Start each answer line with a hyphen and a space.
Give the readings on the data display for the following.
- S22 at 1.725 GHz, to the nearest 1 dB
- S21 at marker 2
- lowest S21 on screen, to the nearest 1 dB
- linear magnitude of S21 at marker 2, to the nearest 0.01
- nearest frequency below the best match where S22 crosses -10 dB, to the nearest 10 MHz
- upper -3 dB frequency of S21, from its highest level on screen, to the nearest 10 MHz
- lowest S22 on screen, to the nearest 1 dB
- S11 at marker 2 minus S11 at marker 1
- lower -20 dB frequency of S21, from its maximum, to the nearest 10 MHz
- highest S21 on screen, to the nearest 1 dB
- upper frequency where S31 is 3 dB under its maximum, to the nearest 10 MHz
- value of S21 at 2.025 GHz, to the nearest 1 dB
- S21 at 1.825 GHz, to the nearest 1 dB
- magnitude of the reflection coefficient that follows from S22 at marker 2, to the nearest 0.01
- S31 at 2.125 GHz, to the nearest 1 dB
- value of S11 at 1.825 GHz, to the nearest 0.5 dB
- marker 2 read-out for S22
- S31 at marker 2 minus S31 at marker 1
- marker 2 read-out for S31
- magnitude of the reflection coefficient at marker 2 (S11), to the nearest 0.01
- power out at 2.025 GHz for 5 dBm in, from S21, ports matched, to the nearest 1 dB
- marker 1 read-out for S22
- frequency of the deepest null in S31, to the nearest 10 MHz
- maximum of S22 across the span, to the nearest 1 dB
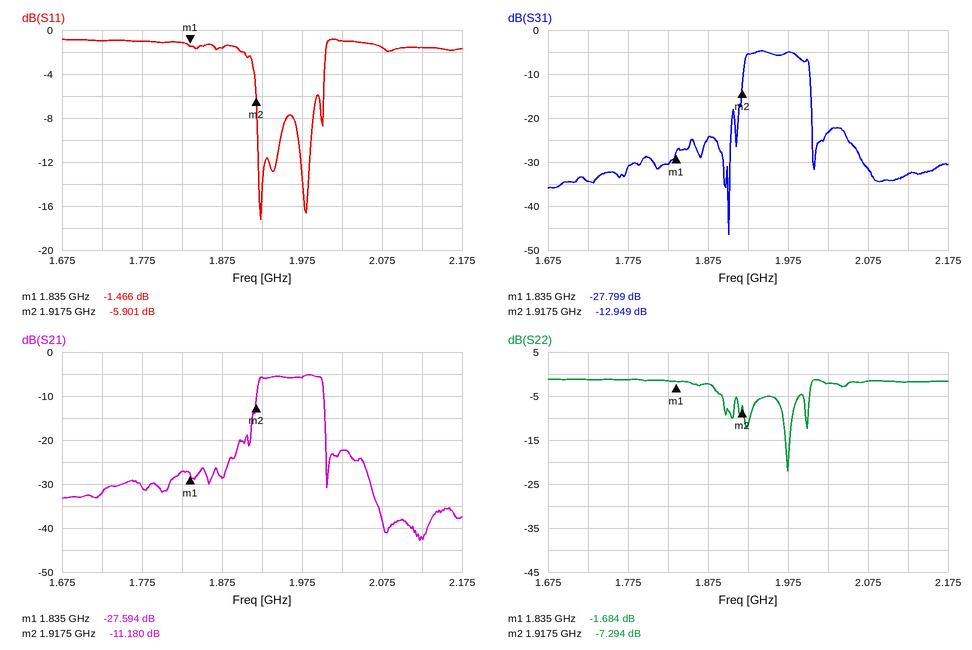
- -1 dB
- -11.180 dB
- -43 dB
- 0.28
- 1.97 GHz
- 2.00 GHz
- -22 dB
- -4.435 dB
- 1.88 GHz
- -5 dB
- 2.00 GHz
- -22 dB
- -27 dB
- 0.43
- -33 dB
- -1.0 dB
- -7.294 dB
- 14.850 dB
- -12.949 dB
- 0.51
- -17 dBm
- -1.684 dB
- 1.90 GHz
- -1 dB
